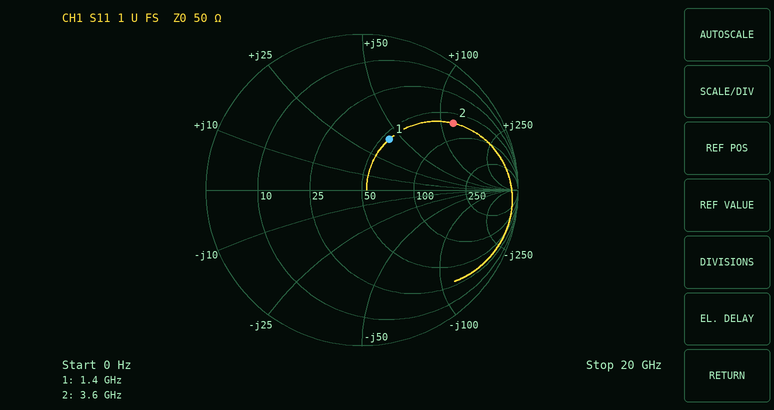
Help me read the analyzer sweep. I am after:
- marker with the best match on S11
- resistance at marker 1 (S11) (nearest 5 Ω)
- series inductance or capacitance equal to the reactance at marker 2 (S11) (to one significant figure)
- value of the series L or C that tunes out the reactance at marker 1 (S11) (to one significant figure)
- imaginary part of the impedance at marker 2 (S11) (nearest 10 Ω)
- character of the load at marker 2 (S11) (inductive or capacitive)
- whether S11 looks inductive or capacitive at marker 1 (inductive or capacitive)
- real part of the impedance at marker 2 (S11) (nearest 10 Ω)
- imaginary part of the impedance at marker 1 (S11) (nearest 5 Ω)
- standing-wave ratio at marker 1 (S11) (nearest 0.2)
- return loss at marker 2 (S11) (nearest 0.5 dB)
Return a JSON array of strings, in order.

["marker 1", "55 Ω", "5 nH", "3 pF", "+120 Ω", "inductive", "inductive", "70 Ω", "+40 Ω", "2.2", "3.0 dB"]
